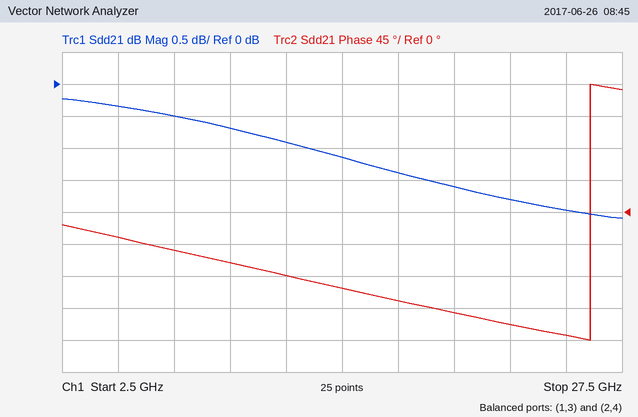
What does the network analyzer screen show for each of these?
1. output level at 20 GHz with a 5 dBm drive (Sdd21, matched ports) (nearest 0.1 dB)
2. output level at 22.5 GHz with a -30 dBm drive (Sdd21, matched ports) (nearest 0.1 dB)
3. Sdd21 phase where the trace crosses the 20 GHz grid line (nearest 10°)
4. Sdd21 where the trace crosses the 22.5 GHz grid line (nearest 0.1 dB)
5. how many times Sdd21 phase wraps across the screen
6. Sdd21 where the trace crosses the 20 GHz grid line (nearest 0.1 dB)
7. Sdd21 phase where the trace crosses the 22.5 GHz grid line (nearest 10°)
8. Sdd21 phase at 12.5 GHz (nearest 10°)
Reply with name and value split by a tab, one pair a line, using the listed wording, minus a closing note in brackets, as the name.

output level at 20 GHz with a 5 dBm drive (Sdd21, matched ports)	3.4 dBm
output level at 22.5 GHz with a -30 dBm drive (Sdd21, matched ports)	-31.8 dBm
Sdd21 phase where the trace crosses the 20 GHz grid line	-140°
Sdd21 where the trace crosses the 22.5 GHz grid line	-1.8 dB
how many times Sdd21 phase wraps across the screen	1
Sdd21 where the trace crosses the 20 GHz grid line	-1.6 dB
Sdd21 phase where the trace crosses the 22.5 GHz grid line	-160°
Sdd21 phase at 12.5 GHz	-90°
